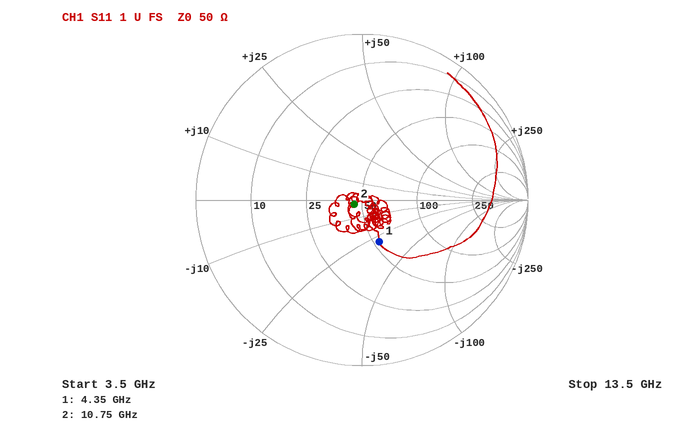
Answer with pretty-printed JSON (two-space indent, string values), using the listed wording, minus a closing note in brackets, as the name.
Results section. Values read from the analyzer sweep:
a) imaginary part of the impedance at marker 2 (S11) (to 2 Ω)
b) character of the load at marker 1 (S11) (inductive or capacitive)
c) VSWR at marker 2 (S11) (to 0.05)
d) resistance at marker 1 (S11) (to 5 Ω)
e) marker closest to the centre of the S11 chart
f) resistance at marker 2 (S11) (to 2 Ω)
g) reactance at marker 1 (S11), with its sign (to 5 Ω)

{
  "imaginary part of the impedance at marker 2 (S11)": "-2 Ω",
  "character of the load at marker 1 (S11)": "capacitive",
  "VSWR at marker 2 (S11)": "1.10",
  "resistance at marker 1 (S11)": "55 Ω",
  "marker closest to the centre of the S11 chart": "marker 2",
  "resistance at marker 2 (S11)": "46 Ω",
  "reactance at marker 1 (S11), with its sign": "-30 Ω"
}
